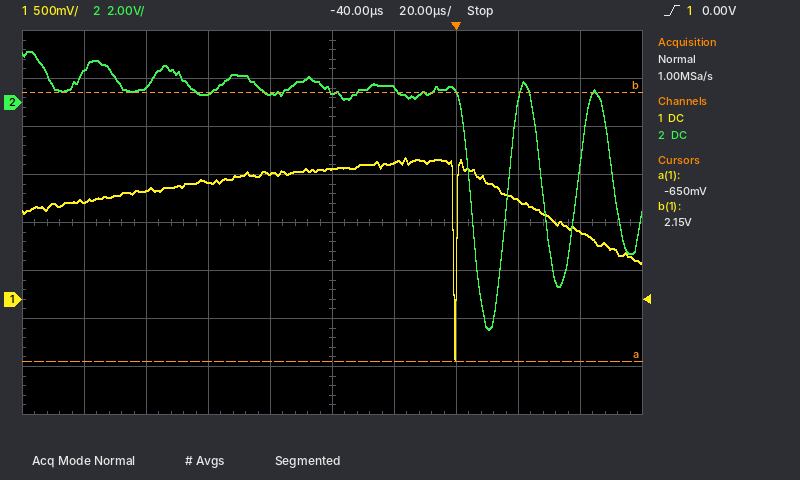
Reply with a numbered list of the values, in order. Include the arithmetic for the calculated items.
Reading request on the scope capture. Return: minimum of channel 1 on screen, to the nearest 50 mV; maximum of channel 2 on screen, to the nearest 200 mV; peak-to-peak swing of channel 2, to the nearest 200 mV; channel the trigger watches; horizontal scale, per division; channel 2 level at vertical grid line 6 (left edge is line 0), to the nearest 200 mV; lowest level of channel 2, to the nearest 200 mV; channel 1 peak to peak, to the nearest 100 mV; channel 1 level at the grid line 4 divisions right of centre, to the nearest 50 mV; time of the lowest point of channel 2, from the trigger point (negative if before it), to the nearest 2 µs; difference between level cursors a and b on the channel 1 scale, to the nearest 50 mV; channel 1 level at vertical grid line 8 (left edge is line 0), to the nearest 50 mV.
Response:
1. -650 mV
2. 2.2 V
3. 2.2 V − (-9.4 V) = 11.6 V
4. channel 1
5. 20 µs
6. 600 mV
7. -9.4 V
8. 2.10 V
9. 700 mV
10. +10 µs
11. 2.80 V
12. 1.05 V
